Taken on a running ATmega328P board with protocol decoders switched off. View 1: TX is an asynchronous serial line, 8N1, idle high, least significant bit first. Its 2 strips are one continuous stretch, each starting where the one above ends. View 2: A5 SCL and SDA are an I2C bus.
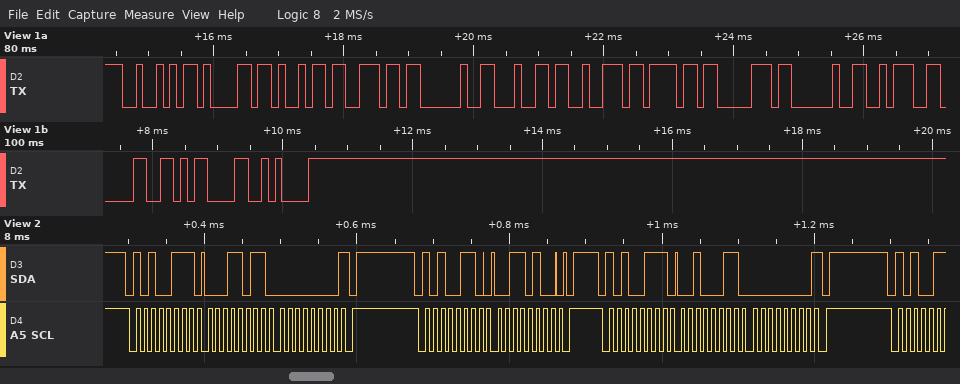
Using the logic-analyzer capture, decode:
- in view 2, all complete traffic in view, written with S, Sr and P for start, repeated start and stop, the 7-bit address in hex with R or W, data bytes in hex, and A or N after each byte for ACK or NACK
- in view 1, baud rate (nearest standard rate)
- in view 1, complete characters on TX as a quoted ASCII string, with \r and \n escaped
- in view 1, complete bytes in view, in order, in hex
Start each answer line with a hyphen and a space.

- S 53R A 1B A 00 N P S 53W A 34 A P S 53R A 23 A 00 N P
- 9600 baud
- "Rain drop :0\r\n"
- 52 61 69 6E 20 64 72 6F 70 20 3A 30 0D 0A
